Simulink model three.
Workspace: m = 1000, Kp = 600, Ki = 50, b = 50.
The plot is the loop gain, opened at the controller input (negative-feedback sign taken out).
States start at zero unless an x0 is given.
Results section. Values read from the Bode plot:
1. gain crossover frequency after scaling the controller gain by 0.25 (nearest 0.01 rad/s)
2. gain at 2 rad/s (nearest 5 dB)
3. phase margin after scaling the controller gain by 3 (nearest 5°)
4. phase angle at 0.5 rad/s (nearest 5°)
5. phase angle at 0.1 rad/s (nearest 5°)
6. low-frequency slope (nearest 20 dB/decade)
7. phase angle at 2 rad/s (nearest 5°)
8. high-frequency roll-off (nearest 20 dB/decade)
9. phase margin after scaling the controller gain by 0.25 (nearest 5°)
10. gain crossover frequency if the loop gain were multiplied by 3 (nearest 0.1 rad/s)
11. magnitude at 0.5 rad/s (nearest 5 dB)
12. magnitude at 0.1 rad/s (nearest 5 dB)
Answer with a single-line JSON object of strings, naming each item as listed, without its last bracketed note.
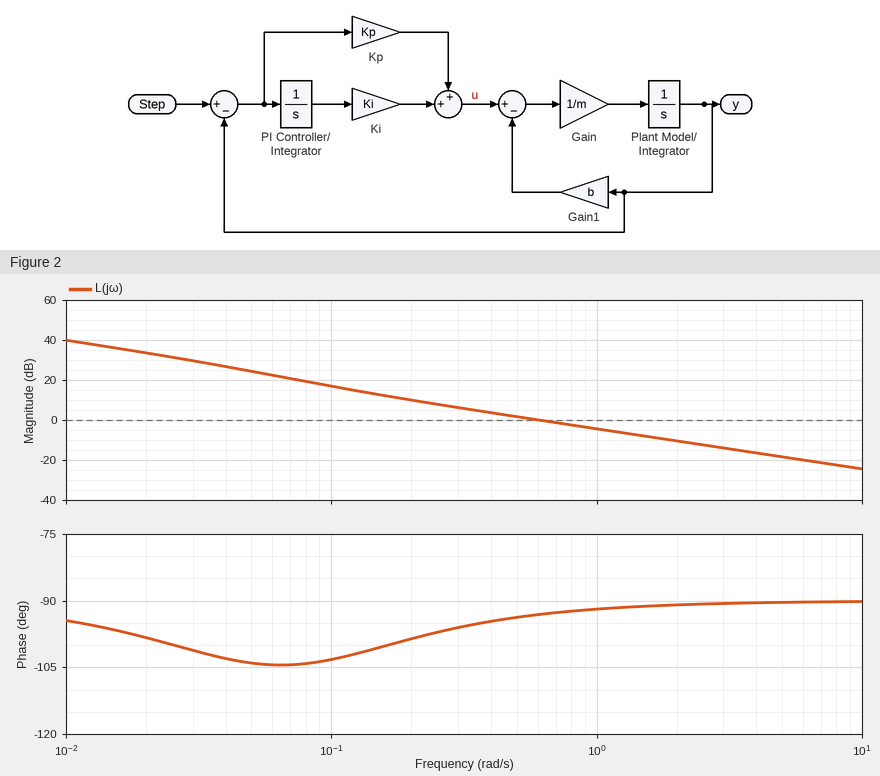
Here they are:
{"gain crossover frequency after scaling the controller gain by 0.25": "0.16 rad/s", "gain at 2 rad/s": "-10 dB", "phase margin after scaling the controller gain by 3": "90°", "phase angle at 0.5 rad/s": "-95°", "phase angle at 0.1 rad/s": "-105°", "low-frequency slope": "-20 dB/decade", "phase angle at 2 rad/s": "-90°", "high-frequency roll-off": "-20 dB/decade", "phase margin after scaling the controller gain by 0.25": "80°", "gain crossover frequency if the loop gain were multiplied by 3": "1.8 rad/s", "magnitude at 0.5 rad/s": "0 dB", "magnitude at 0.1 rad/s": "15 dB"}
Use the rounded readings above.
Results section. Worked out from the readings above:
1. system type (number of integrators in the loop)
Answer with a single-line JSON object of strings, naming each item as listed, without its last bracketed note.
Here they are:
{"system type": "1"}
